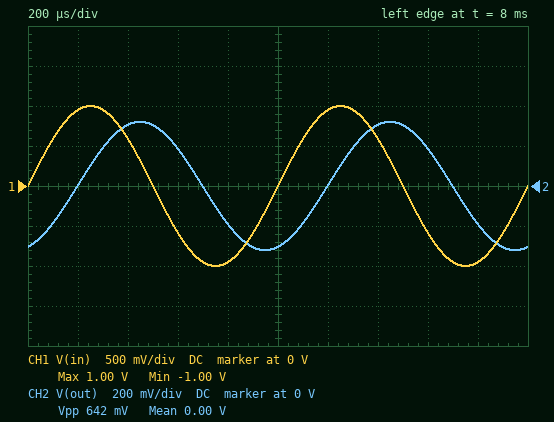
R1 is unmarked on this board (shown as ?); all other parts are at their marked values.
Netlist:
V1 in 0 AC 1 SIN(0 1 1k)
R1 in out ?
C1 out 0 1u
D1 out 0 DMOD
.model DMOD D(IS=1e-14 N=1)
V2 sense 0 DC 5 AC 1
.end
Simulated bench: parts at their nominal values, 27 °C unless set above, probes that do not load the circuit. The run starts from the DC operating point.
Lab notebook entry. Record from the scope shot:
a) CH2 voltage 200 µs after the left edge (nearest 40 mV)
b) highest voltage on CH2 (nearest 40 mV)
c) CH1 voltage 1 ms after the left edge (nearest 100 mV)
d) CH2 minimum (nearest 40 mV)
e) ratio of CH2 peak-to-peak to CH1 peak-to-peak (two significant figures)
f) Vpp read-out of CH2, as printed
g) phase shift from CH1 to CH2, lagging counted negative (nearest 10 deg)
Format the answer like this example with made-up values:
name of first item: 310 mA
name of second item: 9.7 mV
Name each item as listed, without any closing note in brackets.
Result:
CH2 voltage 200 µs after the left edge: 0 V
highest voltage on CH2: 320 mV
CH1 voltage 1 ms after the left edge: 0 V
CH2 minimum: -320 mV
ratio of CH2 peak-to-peak to CH1 peak-to-peak: 0.32
Vpp read-out of CH2, as printed: 642 mV
phase shift from CH1 to CH2, lagging counted negative: -70 deg
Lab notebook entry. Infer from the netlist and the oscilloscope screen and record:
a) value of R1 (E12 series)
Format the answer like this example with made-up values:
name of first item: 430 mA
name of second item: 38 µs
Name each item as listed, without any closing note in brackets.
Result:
value of R1: 470 Ω
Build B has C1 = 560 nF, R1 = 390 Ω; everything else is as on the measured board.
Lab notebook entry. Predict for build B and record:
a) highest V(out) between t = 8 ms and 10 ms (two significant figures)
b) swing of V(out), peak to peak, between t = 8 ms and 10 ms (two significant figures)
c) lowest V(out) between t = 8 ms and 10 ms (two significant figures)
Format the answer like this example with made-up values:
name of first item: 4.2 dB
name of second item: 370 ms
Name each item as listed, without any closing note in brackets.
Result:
highest V(out) between t = 8 ms and 10 ms: 580 mV
swing of V(out), peak to peak, between t = 8 ms and 10 ms: 1.2 V
lowest V(out) between t = 8 ms and 10 ms: -590 mV
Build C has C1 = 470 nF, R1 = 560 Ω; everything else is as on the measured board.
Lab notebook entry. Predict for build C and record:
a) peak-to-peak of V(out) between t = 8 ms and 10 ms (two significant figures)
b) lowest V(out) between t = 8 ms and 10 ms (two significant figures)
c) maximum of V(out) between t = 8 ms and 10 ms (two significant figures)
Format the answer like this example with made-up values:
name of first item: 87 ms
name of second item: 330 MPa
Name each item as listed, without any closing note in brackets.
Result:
peak-to-peak of V(out) between t = 8 ms and 10 ms: 1.0 V
lowest V(out) between t = 8 ms and 10 ms: -520 mV
maximum of V(out) between t = 8 ms and 10 ms: 520 mV
